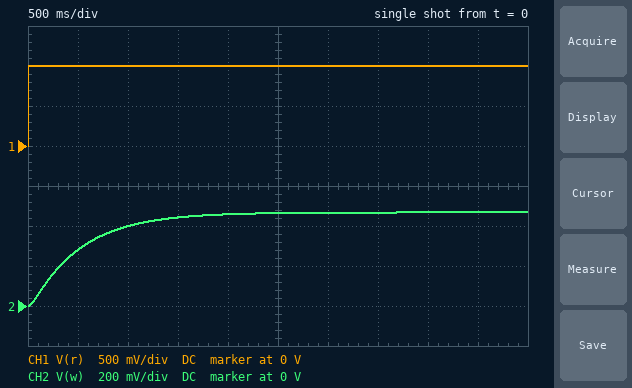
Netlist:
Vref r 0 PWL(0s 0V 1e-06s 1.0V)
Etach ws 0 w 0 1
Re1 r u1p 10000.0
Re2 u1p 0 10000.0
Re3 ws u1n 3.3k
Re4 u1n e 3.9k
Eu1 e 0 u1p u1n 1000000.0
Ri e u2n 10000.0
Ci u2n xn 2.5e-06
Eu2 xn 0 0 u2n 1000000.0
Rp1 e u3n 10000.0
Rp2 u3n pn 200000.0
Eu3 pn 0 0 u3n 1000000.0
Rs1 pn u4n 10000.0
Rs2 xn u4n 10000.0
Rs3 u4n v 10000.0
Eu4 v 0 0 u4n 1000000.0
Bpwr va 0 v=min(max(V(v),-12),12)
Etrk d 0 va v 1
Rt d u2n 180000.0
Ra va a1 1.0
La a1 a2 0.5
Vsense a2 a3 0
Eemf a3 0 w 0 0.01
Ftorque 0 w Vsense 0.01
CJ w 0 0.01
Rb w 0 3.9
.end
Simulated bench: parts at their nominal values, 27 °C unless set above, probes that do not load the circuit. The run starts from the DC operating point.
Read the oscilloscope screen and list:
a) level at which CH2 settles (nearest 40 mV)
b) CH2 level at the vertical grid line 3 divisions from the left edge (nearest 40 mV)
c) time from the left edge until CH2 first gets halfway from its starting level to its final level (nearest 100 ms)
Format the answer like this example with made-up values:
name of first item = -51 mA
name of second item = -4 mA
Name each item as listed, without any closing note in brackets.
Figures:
level at which CH2 settles = 480 mV
CH2 level at the vertical grid line 3 divisions from the left edge = 440 mV
time from the left edge until CH2 first gets halfway from its starting level to its final level = 400 ms
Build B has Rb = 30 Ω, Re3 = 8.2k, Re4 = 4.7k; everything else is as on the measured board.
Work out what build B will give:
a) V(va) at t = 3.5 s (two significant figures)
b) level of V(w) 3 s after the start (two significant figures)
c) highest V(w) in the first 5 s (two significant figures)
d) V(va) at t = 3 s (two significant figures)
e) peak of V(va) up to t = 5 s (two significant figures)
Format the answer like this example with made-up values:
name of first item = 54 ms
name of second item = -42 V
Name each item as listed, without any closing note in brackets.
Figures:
V(va) at t = 3.5 s = 4.6 V
level of V(w) 3 s after the start = 1.4 V
highest V(w) in the first 5 s = 1.7 V
V(va) at t = 3 s = 4.7 V
peak of V(va) up to t = 5 s = 12 V
